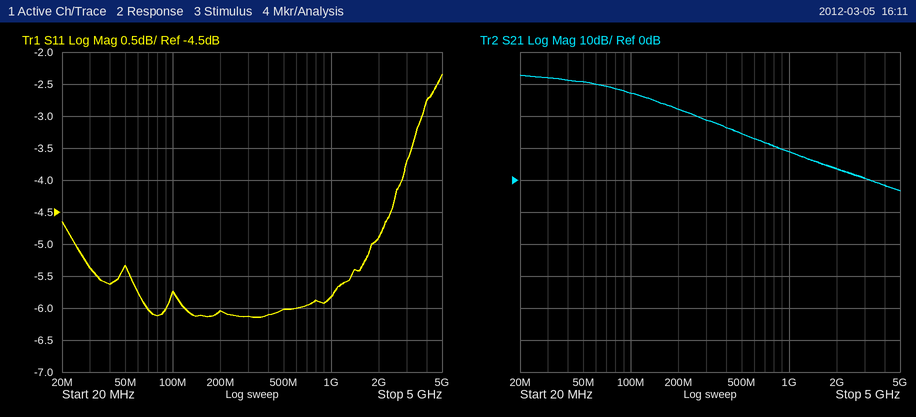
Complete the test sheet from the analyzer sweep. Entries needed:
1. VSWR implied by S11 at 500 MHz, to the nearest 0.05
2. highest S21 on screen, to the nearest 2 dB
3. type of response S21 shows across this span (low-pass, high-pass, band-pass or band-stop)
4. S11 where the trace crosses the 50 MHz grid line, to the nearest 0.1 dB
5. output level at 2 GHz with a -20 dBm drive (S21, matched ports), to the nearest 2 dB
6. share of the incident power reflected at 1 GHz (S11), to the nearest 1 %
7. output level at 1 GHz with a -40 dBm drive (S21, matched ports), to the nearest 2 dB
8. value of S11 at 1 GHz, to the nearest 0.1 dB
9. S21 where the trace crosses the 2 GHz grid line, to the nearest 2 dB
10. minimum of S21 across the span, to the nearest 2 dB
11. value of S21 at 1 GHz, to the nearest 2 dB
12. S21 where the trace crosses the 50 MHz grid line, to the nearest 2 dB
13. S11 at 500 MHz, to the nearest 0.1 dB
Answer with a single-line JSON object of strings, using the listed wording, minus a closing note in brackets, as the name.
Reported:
{"VSWR implied by S11 at 500 MHz, to the nearest 0.05": "3.00", "highest S21 on screen, to the nearest 2 dB": "32 dB", "type of response S21 shows across this span": "low-pass", "S11 where the trace crosses the 50 MHz grid line, to the nearest 0.1 dB": "-5.3 dB", "output level at 2 GHz with a -20 dBm drive (S21, matched ports), to the nearest 2 dB": "-16 dBm", "share of the incident power reflected at 1 GHz (S11), to the nearest 1 %": "26 %", "output level at 1 GHz with a -40 dBm drive (S21, matched ports), to the nearest 2 dB": "-32 dBm", "value of S11 at 1 GHz, to the nearest 0.1 dB": "-5.8 dB", "S21 where the trace crosses the 2 GHz grid line, to the nearest 2 dB": "4 dB", "minimum of S21 across the span, to the nearest 2 dB": "-4 dB", "value of S21 at 1 GHz, to the nearest 2 dB": "8 dB", "S21 where the trace crosses the 50 MHz grid line, to the nearest 2 dB": "30 dB", "S11 at 500 MHz, to the nearest 0.1 dB": "-6.0 dB"}
